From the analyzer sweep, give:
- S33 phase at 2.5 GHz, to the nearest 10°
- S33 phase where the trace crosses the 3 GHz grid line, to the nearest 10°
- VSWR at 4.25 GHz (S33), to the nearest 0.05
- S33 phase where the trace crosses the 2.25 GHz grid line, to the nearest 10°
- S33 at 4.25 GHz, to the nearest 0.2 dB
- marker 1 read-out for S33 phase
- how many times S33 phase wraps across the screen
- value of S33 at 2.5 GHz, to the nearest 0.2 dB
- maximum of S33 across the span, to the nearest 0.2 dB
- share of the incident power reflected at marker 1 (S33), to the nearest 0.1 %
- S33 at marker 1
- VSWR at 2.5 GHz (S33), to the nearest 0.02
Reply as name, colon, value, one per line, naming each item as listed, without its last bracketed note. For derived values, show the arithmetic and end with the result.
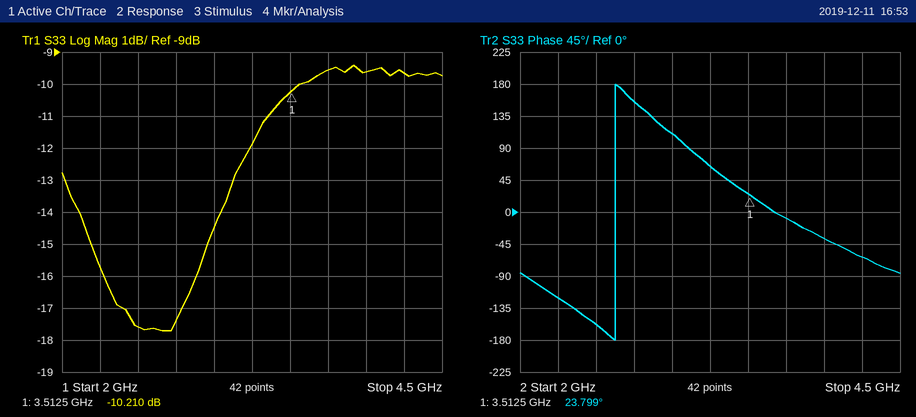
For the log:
S33 phase at 2.5 GHz, to the nearest 10°: -160°
S33 phase where the trace crosses the 3 GHz grid line, to the nearest 10°: 110°
VSWR at 4.25 GHz (S33), to the nearest 0.05: |Γ| = 10^(-9.6/20) = 0.3311; VSWR = (1 + 0.3311)/(1 − 0.3311) ≈ 1.99, so 2.00 to the nearest 0.05
S33 phase where the trace crosses the 2.25 GHz grid line, to the nearest 10°: -120°
S33 at 4.25 GHz, to the nearest 0.2 dB: -9.6 dB
marker 1 read-out for S33 phase: 23.799°
how many times S33 phase wraps across the screen: 1
value of S33 at 2.5 GHz, to the nearest 0.2 dB: -17.6 dB
maximum of S33 across the span, to the nearest 0.2 dB: -9.4 dB
share of the incident power reflected at marker 1 (S33), to the nearest 0.1 %: 10^(-10.21/10) ≈ 9.5 %
S33 at marker 1: -10.210 dB
VSWR at 2.5 GHz (S33), to the nearest 0.02: |Γ| = 10^(-17.6/20) = 0.1318; VSWR = (1 + 0.1318)/(1 − 0.1318) ≈ 1.30
